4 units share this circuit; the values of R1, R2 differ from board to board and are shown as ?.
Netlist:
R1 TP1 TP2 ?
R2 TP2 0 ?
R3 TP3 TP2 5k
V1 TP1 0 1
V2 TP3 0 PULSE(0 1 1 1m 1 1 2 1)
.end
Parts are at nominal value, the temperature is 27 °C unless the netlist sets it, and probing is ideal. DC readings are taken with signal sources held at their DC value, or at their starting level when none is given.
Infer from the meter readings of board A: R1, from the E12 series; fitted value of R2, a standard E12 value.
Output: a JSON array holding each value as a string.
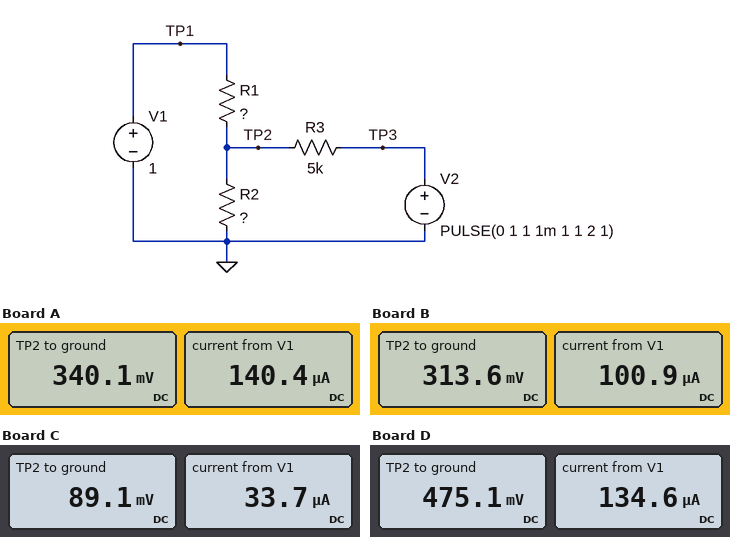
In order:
["4.7 kΩ", "4.7 kΩ"]
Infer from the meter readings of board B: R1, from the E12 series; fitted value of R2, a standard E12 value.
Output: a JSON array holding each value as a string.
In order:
["6.8 kΩ", "8.2 kΩ"]
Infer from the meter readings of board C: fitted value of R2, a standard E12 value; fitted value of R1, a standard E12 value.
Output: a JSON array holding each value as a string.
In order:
["5.6 kΩ", "27 kΩ"]
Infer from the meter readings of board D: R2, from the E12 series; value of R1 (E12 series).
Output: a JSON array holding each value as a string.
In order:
["12 kΩ", "3.9 kΩ"]
